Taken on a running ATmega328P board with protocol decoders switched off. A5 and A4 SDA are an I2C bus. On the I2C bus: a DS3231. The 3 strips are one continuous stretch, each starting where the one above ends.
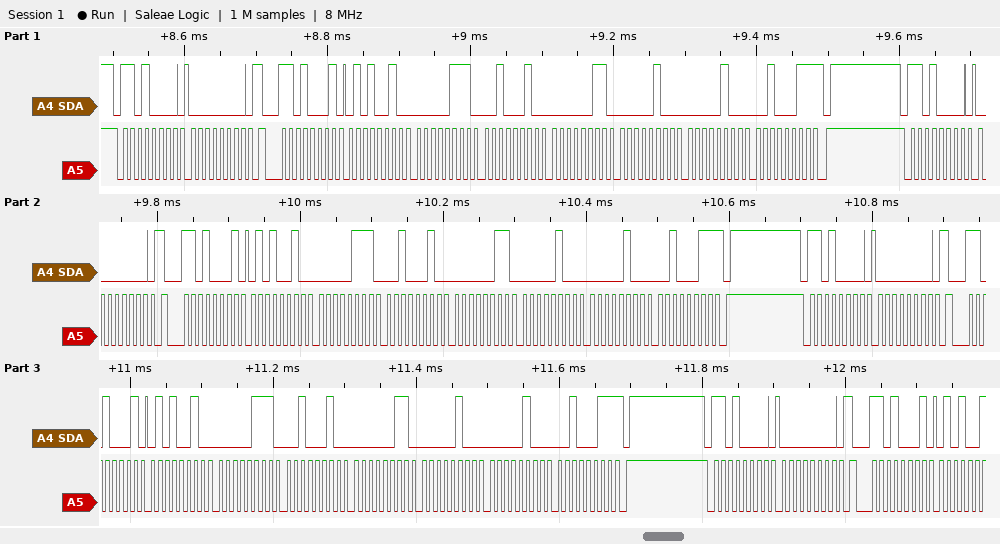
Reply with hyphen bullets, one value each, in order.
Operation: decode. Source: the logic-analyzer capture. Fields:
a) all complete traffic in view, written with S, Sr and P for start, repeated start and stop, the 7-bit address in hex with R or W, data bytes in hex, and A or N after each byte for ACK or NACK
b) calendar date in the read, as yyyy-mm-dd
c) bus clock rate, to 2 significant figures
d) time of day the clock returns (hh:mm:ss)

- S 68W A 00 A Sr 68R A 52 A 07 A 22 A 03 A 04 A 04 A 23 N P S 68W A 00 A Sr 68R A 52 A 07 A 22 A 03 A 04 A 04 A 23 N P S 68W A 00 A Sr 68R A 52 A 07 A 22 A 03 A 04 A 04 A 23 N P S 68W A 00 A Sr 68R A
- 2023-04-04
- 100 kHz
- 22:07:52
